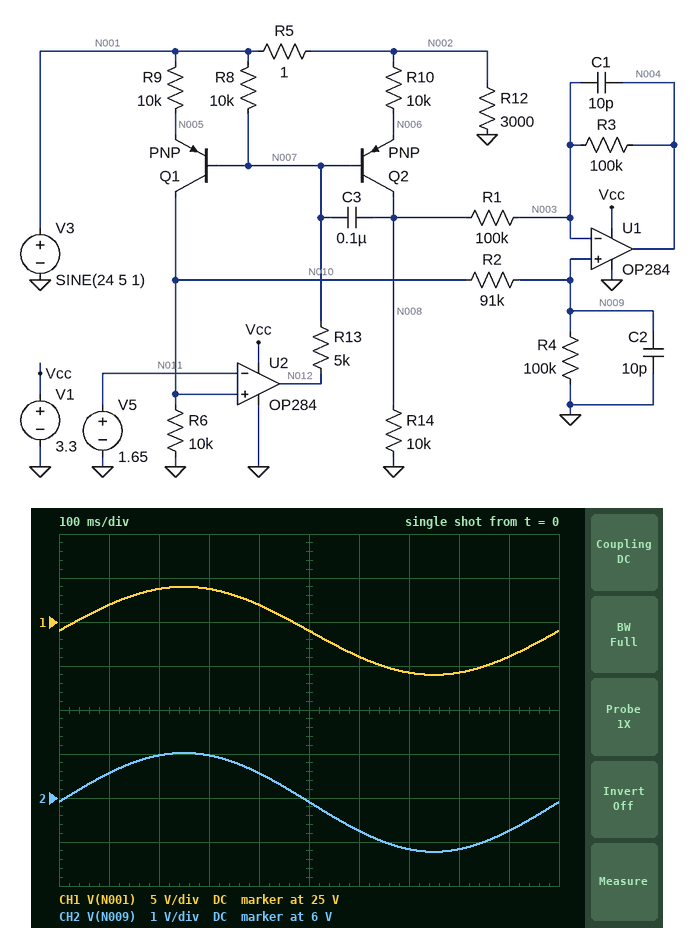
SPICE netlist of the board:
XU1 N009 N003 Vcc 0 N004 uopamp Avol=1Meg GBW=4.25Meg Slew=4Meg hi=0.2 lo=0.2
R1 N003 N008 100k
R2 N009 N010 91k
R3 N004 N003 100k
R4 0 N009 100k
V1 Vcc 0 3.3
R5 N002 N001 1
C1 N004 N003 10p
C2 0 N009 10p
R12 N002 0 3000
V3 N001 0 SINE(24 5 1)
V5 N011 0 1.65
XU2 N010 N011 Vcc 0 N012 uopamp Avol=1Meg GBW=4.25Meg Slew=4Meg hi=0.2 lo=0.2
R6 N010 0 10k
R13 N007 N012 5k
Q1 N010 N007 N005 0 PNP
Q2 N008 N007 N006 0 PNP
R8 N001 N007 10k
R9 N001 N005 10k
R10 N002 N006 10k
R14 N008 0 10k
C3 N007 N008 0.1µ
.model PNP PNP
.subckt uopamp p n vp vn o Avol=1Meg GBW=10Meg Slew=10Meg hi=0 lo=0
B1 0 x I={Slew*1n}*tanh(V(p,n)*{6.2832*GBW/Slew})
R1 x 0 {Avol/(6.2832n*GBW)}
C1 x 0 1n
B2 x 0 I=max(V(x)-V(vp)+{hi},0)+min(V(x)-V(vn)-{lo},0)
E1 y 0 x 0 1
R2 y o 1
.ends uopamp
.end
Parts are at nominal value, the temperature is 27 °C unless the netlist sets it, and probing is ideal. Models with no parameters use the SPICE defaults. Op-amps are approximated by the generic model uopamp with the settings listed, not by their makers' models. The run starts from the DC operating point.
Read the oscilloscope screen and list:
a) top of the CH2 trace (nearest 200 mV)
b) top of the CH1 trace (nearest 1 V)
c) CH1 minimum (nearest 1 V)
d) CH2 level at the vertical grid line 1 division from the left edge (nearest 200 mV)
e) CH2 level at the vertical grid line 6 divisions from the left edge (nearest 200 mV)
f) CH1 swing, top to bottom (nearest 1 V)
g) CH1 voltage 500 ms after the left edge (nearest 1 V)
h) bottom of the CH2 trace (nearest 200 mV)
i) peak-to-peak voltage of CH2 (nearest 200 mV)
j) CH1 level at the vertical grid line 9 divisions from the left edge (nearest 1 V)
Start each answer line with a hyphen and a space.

- 7.0 V
- 29 V
- 19 V
- 6.6 V
- 5.2 V
- 10 V
- 24 V
- 4.8 V
- 2.2 V
- 21 V
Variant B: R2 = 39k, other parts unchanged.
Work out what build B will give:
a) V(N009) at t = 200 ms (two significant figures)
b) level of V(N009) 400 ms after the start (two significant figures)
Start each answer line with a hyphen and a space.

- 9.6 V
- 9.0 V
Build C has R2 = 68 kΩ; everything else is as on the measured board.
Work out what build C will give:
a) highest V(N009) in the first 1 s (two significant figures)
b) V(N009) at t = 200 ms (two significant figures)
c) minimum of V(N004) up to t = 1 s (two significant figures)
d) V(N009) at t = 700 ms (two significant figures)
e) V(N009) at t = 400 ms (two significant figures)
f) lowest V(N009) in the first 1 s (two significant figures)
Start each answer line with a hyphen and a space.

- 8.0 V
- 7.9 V
- 1.7 V
- 5.5 V
- 7.5 V
- 5.4 V
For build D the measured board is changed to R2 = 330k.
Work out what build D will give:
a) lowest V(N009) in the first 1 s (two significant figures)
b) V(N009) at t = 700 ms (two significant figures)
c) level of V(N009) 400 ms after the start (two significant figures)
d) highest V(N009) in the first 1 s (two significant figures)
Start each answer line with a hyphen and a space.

- 2.1 V
- 2.2 V
- 2.9 V
- 3.1 V
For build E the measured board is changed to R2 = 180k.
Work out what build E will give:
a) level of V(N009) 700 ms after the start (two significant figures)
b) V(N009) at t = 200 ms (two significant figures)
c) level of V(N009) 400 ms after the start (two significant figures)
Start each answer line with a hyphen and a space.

- 3.3 V
- 4.8 V
- 4.5 V
